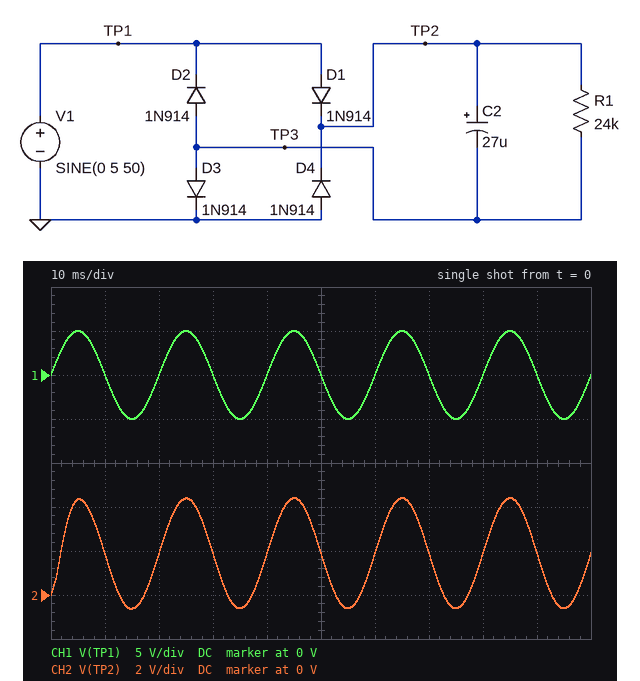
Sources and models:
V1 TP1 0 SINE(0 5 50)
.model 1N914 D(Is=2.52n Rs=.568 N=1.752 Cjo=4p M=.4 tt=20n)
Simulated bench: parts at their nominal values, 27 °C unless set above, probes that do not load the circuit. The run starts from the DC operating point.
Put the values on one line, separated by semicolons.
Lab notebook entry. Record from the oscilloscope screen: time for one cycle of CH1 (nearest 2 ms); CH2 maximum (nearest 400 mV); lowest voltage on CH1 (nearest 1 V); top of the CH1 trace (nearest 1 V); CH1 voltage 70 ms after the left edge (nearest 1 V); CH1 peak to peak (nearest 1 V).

20 ms; 4.4 V; -5 V; 5 V; 0 V; 10 V
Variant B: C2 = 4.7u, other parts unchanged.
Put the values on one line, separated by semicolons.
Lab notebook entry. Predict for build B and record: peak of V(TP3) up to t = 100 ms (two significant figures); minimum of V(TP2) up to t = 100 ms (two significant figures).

680 mV; -600 mV
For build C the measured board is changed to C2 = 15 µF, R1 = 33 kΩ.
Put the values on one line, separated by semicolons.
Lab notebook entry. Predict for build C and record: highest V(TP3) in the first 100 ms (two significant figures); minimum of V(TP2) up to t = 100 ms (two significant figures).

740 mV; -600 mV
